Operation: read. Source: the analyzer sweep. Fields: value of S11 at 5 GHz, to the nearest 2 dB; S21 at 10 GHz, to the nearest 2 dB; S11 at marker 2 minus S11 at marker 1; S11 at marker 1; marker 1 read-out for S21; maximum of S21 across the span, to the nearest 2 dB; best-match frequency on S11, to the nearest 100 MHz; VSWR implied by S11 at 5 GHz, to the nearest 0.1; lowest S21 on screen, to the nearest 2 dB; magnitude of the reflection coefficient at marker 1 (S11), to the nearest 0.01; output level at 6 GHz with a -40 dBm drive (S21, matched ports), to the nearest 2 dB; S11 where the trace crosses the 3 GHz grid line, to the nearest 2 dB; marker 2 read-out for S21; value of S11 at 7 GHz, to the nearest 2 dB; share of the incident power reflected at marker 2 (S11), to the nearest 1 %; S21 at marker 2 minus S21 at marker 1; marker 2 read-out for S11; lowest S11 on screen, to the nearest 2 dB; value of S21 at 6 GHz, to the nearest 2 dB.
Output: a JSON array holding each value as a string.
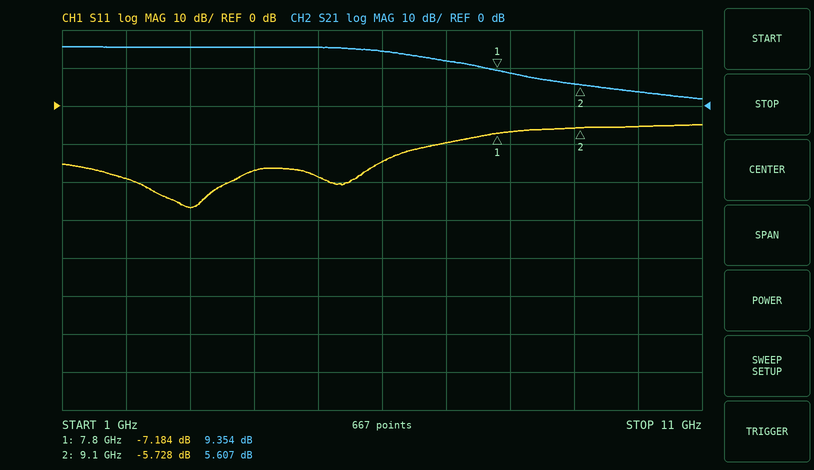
["-18 dB", "4 dB", "1.456 dB", "-7.184 dB", "9.354 dB", "16 dB", "3.0 GHz", "1.3", "2 dB", "0.44", "-26 dBm", "-26 dB", "5.607 dB", "-10 dB", "27 %", "-3.747 dB", "-5.728 dB", "-26 dB", "14 dB"]
